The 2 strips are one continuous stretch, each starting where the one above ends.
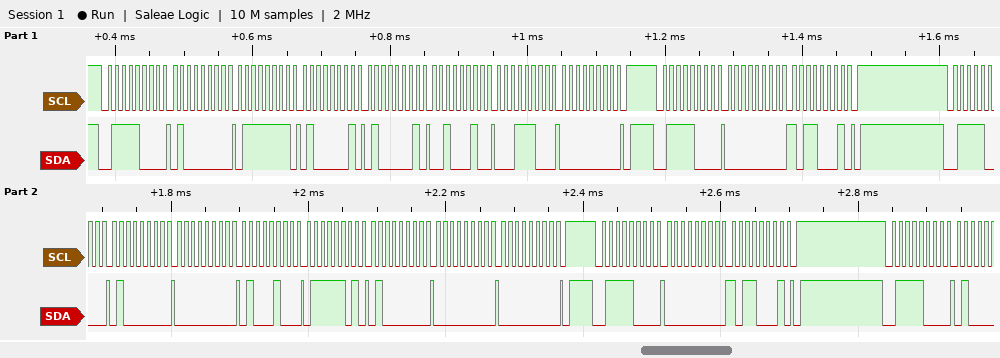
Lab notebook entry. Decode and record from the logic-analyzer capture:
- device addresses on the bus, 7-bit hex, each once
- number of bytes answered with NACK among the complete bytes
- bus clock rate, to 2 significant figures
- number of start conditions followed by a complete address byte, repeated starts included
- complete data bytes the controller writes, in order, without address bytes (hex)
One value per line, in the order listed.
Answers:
0x3C
0
100 kHz
5
40 7F 41 41 22 1C 00 00 B1 40 00 44 7D 40 00 00 00 B1
